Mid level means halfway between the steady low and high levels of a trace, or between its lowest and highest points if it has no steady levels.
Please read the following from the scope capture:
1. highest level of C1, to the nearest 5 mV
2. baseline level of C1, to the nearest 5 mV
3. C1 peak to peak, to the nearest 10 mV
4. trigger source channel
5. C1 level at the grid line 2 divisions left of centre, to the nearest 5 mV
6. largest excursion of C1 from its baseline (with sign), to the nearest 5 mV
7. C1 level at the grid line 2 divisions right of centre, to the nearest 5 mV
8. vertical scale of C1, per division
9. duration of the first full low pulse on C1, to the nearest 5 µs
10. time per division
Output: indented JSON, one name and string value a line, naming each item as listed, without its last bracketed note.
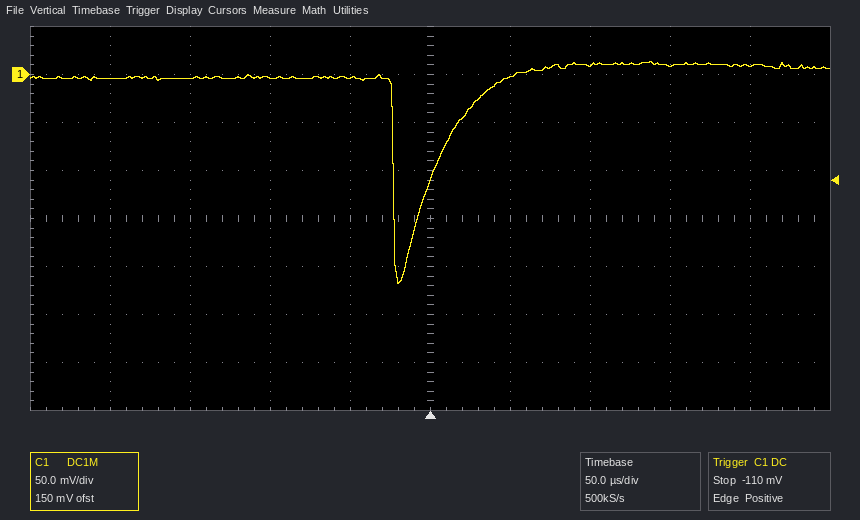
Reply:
{
  "highest level of C1, to the nearest 5 mV": "15 mV",
  "baseline level of C1, to the nearest 5 mV": "-5 mV",
  "C1 peak to peak, to the nearest 10 mV": "230 mV",
  "trigger source channel": "C1",
  "C1 level at the grid line 2 divisions left of centre, to the nearest 5 mV": "-5 mV",
  "largest excursion of C1 from its baseline (with sign), to the nearest 5 mV": "-215 mV",
  "C1 level at the grid line 2 divisions right of centre, to the nearest 5 mV": "10 mV",
  "vertical scale of C1, per division": "50 mV",
  "duration of the first full low pulse on C1, to the nearest 5 µs": "25 µs",
  "time per division": "50 µs"
}
